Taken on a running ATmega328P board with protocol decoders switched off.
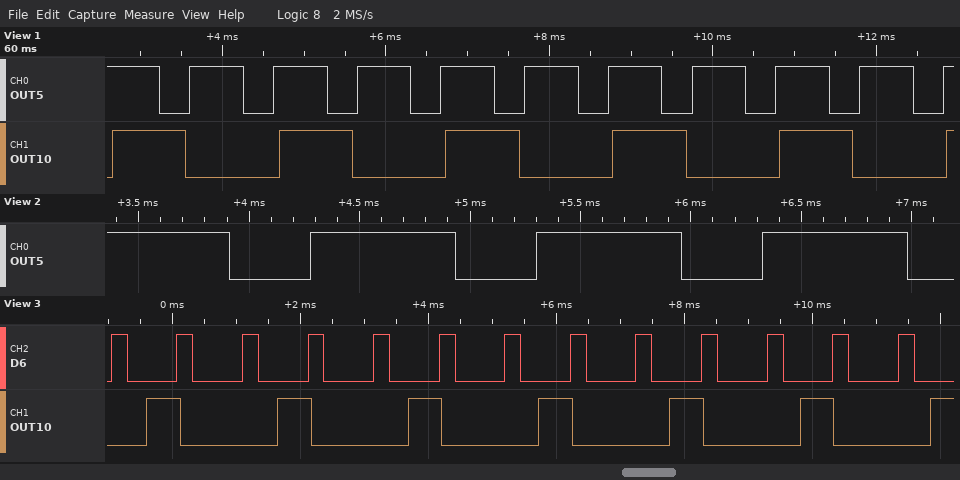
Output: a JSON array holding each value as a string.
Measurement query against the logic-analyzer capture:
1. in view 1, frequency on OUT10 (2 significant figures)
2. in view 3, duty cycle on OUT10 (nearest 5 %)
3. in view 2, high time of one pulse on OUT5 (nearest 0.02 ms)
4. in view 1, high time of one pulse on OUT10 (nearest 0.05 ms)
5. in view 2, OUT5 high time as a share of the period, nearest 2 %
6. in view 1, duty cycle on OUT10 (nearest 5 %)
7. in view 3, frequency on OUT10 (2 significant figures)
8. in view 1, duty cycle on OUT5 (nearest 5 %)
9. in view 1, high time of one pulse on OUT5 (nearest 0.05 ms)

["490 Hz", "25 %", "0.66 ms", "0.90 ms", "64 %", "45 %", "490 Hz", "65 %", "0.65 ms"]
